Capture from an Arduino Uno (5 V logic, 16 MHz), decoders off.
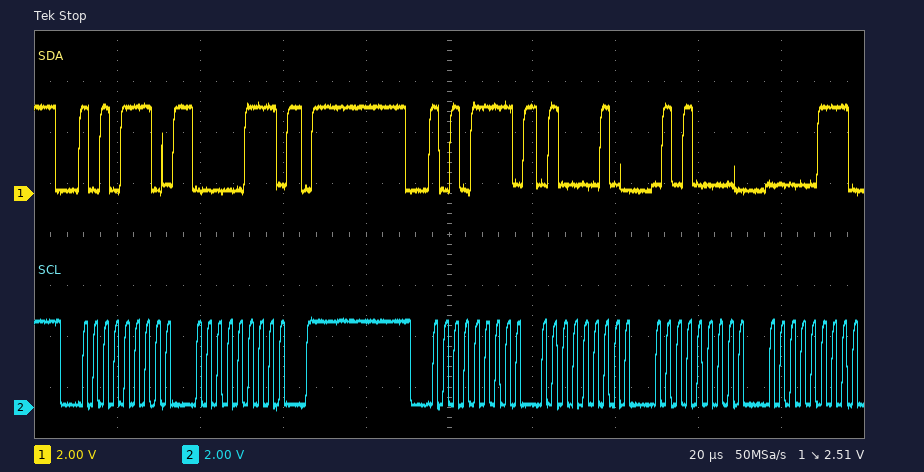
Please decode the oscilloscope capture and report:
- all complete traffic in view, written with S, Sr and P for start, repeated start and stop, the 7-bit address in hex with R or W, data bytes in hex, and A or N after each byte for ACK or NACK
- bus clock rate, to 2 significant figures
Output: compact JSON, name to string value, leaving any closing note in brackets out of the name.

{"all complete traffic in view, written with S, Sr and P for start, repeated start and stop, the 7-bit address in hex with R or W, data bytes in hex, and A or N after each byte for ACK or NACK": "S 57W A 07 A P S 57R A 42 A 50 A 07 A", "bus clock rate, to 2 significant figures": "400 kHz"}
